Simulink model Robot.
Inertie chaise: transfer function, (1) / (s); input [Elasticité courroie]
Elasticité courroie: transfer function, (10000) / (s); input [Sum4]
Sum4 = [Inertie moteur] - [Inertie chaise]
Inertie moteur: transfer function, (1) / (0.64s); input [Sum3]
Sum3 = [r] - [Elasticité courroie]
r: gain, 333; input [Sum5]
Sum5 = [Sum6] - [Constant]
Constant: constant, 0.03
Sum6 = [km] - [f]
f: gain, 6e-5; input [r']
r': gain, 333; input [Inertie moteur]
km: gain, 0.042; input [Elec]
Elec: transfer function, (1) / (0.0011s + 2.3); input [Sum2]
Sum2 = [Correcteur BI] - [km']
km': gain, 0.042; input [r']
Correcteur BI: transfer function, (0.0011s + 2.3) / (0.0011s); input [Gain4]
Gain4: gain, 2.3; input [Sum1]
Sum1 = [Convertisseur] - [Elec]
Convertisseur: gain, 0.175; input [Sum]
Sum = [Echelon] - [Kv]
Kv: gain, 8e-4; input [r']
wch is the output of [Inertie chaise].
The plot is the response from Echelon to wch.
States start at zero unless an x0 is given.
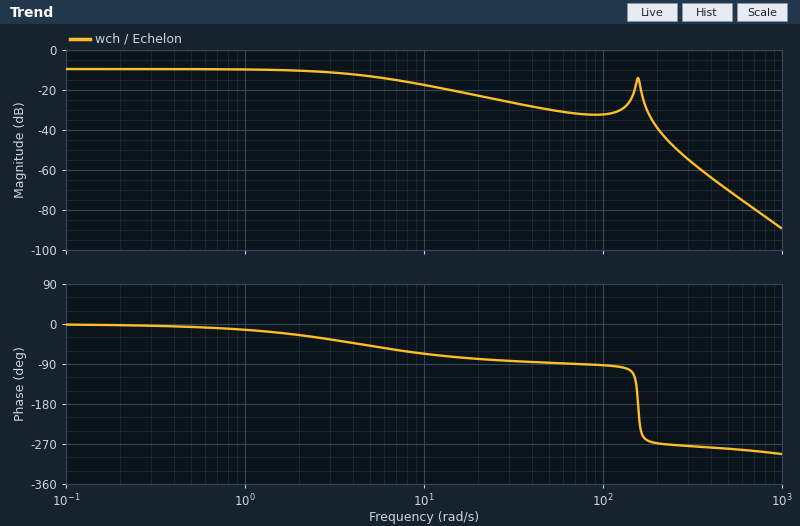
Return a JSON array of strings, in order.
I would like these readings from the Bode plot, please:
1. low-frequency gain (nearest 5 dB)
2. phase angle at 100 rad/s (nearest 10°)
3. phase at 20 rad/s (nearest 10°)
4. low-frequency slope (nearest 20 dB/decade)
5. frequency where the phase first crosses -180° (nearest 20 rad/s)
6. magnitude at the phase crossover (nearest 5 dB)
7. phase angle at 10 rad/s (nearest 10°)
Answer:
["-10 dB", "-90°", "-80°", "0 dB/decade", "160 rad/s", "-15 dB", "-70°"]
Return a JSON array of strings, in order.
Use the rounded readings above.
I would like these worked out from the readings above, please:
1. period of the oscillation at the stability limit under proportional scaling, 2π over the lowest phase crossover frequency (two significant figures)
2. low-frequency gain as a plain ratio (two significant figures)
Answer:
["0.039 s", "0.32"]
